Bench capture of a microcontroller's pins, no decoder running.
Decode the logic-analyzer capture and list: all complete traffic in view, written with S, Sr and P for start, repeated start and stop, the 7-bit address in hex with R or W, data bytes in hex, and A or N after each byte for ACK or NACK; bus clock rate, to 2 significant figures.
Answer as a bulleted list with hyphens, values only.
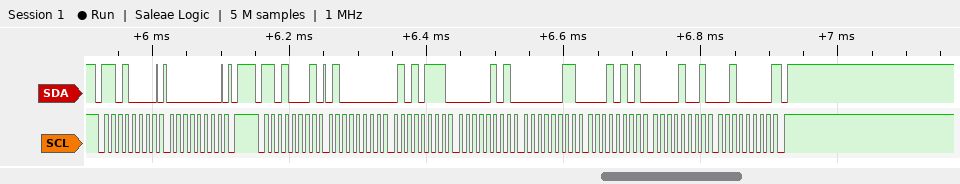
- S 68W A 00 A P S 68R A 40 A 57 A 05 A 03 A 15 A 09 A 20 N P
- 100 kHz
